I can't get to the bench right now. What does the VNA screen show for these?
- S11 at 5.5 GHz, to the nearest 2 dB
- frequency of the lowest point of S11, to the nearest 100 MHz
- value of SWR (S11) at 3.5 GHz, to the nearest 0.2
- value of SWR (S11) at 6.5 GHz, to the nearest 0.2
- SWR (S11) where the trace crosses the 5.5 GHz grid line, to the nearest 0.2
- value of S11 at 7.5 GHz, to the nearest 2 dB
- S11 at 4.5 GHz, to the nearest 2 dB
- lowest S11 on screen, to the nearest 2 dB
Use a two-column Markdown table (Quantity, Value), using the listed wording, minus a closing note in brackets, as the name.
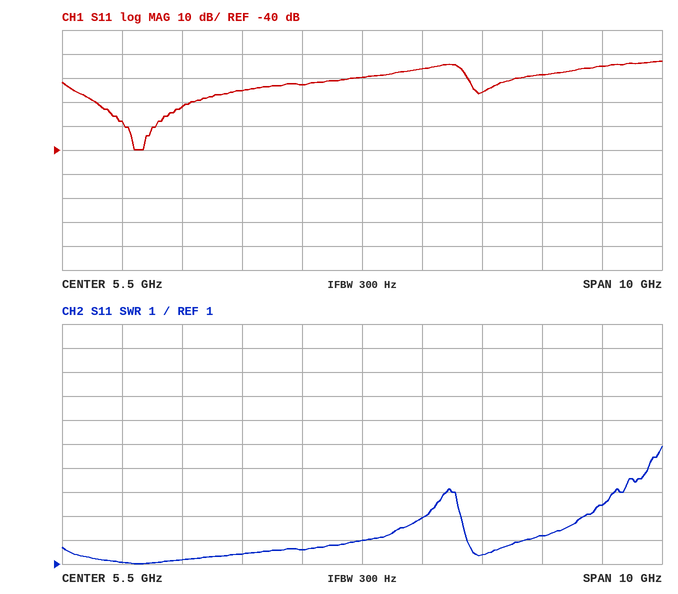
| Quantity | Value |
|---|---|
| S11 at 5.5 GHz, to the nearest 2 dB | -10 dB |
| frequency of the lowest point of S11, to the nearest 100 MHz | 1.7 GHz |
| value of SWR (S11) at 3.5 GHz, to the nearest 0.2 | 1.4 |
| value of SWR (S11) at 6.5 GHz, to the nearest 0.2 | 3.0 |
| SWR (S11) where the trace crosses the 5.5 GHz grid line, to the nearest 0.2 | 2.0 |
| value of S11 at 7.5 GHz, to the nearest 2 dB | -16 dB |
| S11 at 4.5 GHz, to the nearest 2 dB | -12 dB |
| lowest S11 on screen, to the nearest 2 dB | -40 dB |
